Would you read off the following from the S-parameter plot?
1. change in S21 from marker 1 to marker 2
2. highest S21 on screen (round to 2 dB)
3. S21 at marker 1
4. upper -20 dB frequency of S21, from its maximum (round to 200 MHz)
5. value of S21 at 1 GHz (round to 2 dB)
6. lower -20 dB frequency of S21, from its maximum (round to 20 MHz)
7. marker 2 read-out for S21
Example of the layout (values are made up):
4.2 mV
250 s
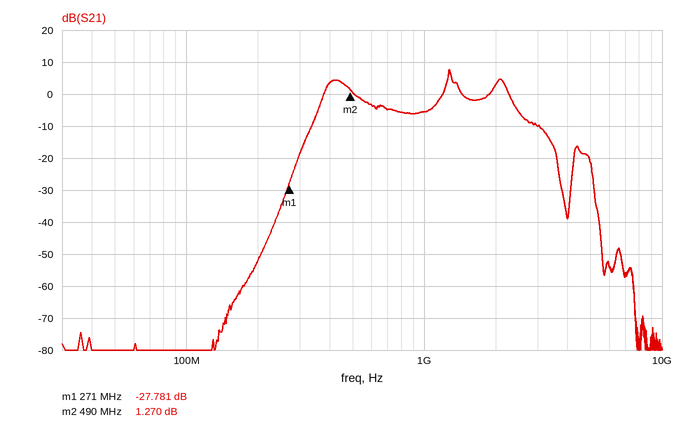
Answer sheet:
29.051 dB
8 dB
-27.781 dB
3.2 GHz
-6 dB
320 MHz
1.270 dB
